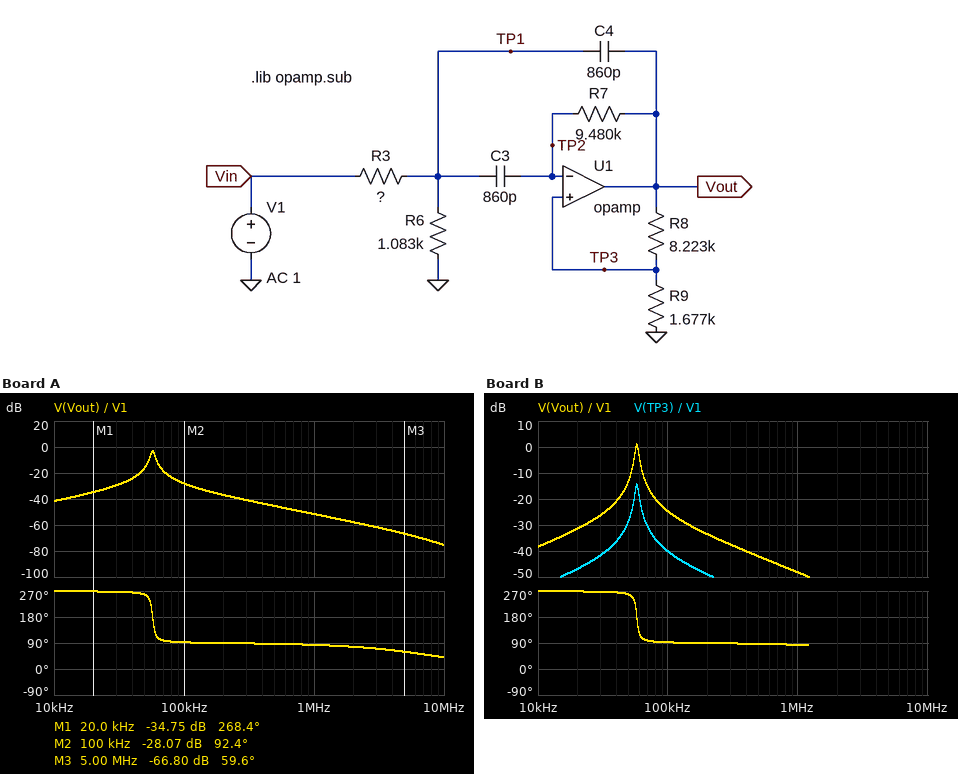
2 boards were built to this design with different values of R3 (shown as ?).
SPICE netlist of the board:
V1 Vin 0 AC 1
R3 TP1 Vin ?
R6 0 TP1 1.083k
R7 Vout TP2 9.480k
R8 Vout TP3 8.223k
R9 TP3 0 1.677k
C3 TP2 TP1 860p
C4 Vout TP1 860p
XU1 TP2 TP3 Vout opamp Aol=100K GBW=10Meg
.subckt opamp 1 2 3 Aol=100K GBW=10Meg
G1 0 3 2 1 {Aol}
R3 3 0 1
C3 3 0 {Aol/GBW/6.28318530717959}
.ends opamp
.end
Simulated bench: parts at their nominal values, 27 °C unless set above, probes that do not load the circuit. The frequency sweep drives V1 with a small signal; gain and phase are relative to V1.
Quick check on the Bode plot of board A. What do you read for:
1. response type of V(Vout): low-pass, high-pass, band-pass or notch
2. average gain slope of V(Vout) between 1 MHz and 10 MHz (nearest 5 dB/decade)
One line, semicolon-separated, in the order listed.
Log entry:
band-pass; -25 dB/decade
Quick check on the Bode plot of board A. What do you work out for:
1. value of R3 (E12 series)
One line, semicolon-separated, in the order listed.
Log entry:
82 kΩ
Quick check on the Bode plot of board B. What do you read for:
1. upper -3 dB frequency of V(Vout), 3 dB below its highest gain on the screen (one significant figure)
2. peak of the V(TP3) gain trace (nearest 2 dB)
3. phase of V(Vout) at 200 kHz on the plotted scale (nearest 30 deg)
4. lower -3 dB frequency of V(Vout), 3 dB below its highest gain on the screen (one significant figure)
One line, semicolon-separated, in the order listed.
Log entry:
60 kHz; -14 dB; 90 deg; 60 kHz
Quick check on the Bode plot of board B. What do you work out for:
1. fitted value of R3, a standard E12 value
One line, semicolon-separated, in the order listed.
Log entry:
56 kΩ
